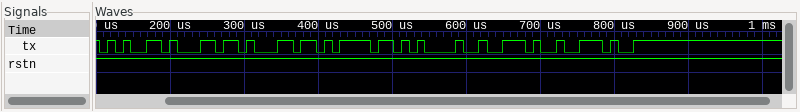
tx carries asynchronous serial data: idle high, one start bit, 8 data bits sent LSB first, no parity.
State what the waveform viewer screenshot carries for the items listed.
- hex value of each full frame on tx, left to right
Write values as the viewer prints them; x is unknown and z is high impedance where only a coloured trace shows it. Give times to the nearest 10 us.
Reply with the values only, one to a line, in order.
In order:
65, 6C, 6C, 6F, 21, 2E, 2E
